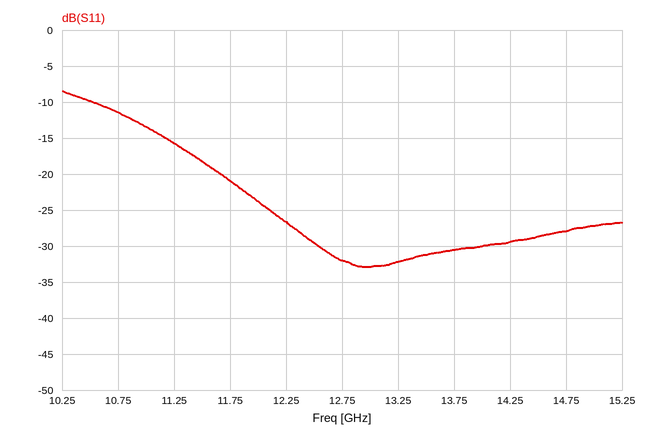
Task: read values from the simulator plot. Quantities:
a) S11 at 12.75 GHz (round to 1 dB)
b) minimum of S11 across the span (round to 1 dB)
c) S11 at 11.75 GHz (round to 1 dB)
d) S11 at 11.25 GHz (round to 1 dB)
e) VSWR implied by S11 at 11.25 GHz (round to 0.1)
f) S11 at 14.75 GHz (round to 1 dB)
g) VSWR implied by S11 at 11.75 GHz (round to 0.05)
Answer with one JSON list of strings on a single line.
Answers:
["-32 dB", "-33 dB", "-21 dB", "-16 dB", "1.4", "-28 dB", "1.20"]
